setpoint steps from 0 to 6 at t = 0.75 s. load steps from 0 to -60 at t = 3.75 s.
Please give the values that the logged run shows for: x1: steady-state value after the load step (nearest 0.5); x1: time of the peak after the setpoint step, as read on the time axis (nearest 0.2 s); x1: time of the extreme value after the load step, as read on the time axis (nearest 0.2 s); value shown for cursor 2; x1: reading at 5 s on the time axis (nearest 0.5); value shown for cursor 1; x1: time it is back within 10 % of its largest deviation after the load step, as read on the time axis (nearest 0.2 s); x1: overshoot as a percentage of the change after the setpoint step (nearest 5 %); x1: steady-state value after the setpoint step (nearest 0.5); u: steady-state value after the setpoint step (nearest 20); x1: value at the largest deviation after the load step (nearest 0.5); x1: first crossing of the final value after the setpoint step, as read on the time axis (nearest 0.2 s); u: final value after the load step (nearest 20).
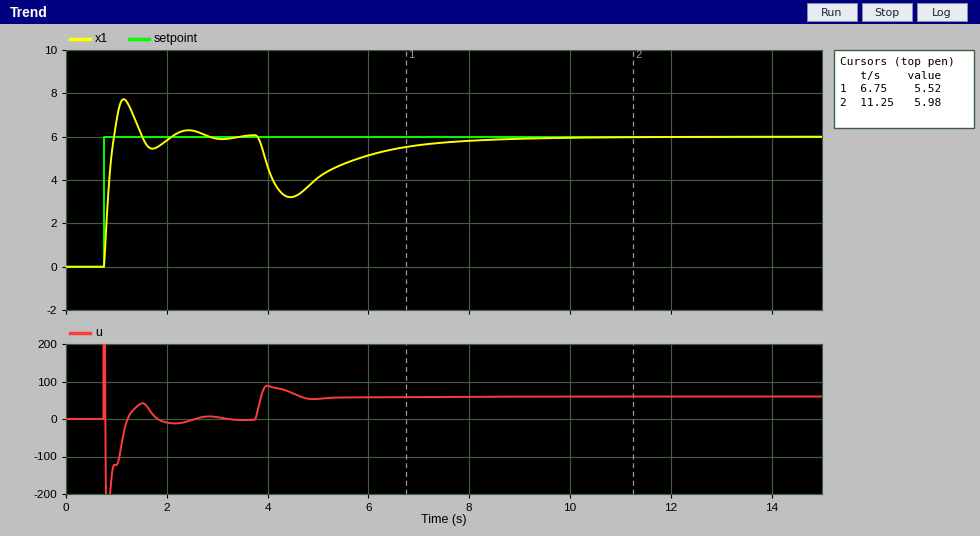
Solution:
6.0
1.2 s
4.4 s
5.98
4.0
5.52
7.4 s
30 %
6.0
0
3.0
1.0 s
60
